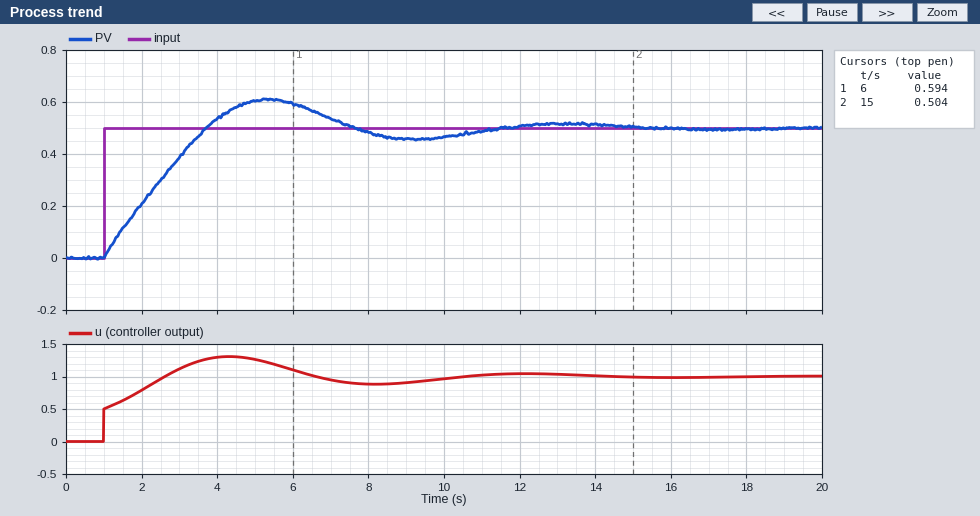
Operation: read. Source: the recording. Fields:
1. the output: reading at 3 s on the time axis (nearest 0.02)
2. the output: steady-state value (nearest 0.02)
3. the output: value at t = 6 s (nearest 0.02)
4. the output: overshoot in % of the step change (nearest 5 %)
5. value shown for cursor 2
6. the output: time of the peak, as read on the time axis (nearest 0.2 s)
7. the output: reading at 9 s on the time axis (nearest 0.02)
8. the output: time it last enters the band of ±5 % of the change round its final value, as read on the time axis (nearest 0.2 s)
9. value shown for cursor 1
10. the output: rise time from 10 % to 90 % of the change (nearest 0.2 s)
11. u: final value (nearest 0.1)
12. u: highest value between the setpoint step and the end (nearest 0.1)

0.38
0.50
0.60
20 %
0.504
5.4 s
0.46
10.4 s
0.594
2.2 s
1.0
1.3
